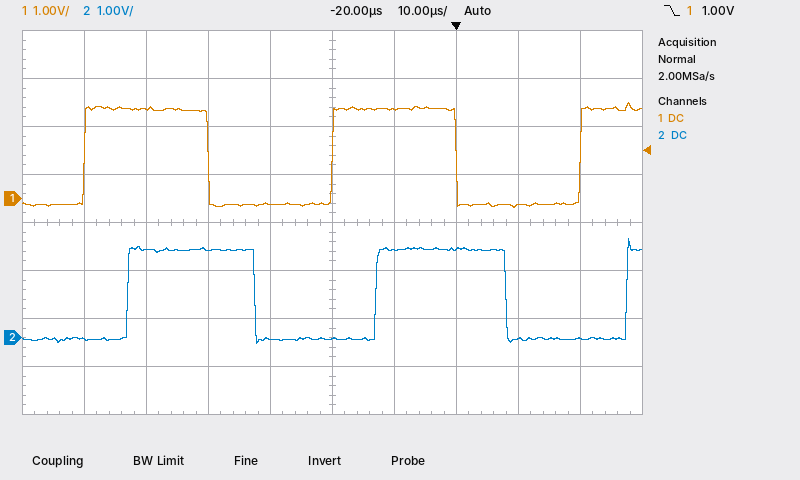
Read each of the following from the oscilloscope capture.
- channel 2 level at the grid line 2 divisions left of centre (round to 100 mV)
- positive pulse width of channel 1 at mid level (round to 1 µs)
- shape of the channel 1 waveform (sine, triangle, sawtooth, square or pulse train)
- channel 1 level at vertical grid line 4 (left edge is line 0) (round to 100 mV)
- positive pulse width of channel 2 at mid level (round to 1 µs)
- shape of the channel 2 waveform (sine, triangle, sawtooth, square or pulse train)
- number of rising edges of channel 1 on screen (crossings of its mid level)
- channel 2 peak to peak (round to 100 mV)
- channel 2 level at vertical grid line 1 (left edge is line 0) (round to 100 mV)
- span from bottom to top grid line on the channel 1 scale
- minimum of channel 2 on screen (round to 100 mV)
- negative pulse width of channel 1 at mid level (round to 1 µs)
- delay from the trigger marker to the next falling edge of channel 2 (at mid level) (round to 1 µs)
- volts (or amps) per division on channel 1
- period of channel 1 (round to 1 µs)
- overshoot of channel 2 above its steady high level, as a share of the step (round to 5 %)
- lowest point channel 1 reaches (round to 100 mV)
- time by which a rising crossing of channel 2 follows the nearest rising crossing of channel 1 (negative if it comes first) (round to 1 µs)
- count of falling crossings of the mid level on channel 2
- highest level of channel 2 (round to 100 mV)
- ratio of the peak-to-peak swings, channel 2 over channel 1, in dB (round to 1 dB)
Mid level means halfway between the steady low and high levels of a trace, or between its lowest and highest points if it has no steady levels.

1.8 V
20 µs
square
-100 mV
21 µs
square
3
2.2 V
0.0 V
8 V
-100 mV
20 µs
8 µs
1 V
40 µs
10 %
-200 mV
+7 µs
2
2.1 V
0 dB
